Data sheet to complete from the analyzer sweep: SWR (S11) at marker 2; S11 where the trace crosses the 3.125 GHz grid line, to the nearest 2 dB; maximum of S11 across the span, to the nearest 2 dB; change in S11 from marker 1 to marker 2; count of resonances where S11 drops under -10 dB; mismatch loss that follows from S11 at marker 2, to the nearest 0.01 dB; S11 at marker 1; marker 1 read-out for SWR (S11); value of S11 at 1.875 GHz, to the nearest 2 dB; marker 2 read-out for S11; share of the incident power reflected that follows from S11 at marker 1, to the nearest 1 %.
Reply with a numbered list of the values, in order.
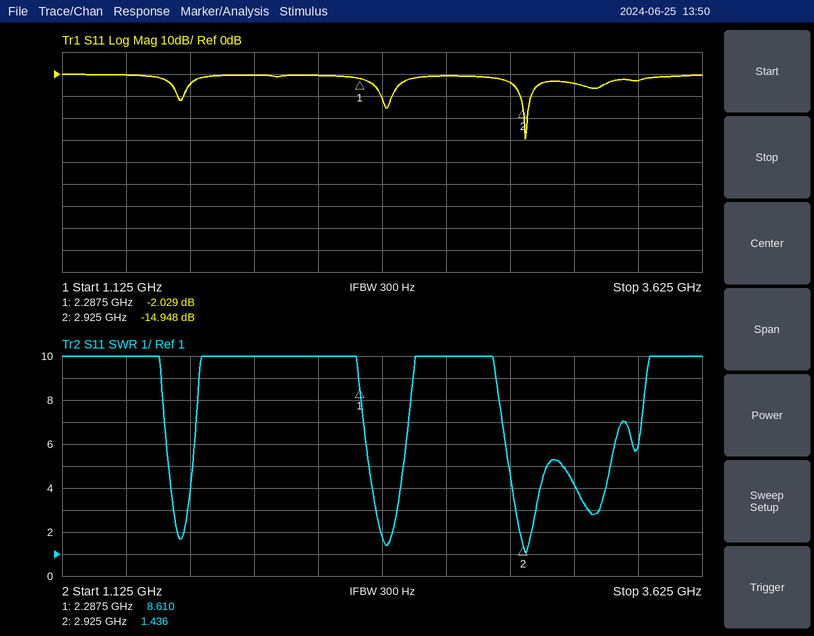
1. 1.436
2. -4 dB
3. 0 dB
4. -12.919 dB
5. 3
6. 0.14 dB
7. -2.029 dB
8. 8.610
9. 0 dB
10. -14.948 dB
11. 63 %
